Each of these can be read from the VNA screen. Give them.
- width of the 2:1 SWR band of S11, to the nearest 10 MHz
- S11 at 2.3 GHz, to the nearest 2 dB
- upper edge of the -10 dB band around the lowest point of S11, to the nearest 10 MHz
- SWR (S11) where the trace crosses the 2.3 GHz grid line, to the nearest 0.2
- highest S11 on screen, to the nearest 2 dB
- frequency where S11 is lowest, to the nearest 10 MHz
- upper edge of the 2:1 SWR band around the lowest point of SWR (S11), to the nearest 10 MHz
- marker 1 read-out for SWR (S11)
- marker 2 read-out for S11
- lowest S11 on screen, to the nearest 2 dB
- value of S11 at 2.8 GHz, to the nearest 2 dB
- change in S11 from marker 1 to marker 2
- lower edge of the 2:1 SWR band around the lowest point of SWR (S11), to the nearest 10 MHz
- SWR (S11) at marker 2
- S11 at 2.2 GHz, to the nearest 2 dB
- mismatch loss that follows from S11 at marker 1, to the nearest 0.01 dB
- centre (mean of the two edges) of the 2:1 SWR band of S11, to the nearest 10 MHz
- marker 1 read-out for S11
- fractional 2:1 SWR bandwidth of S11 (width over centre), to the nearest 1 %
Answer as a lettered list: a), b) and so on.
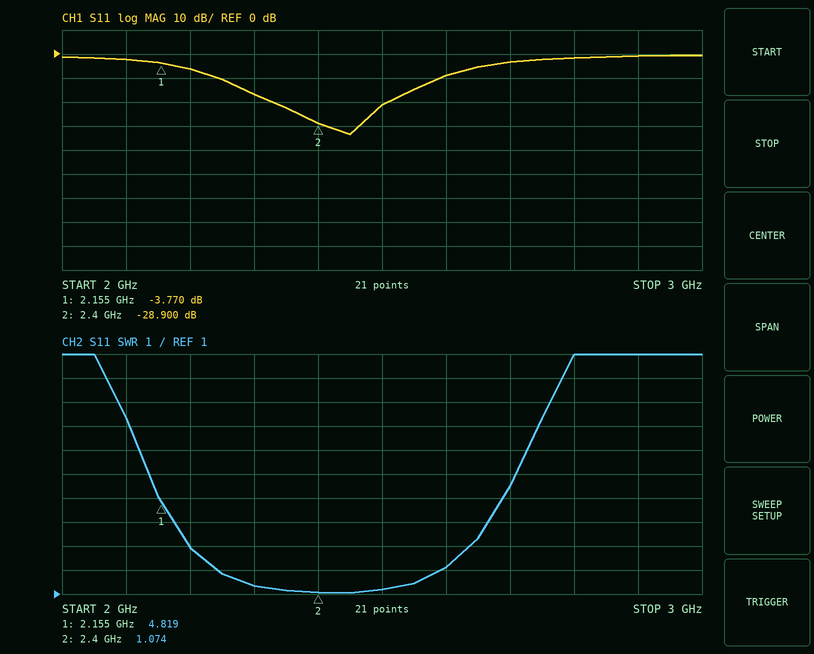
a) 350 MHz
b) -16 dB
c) 2.59 GHz
d) 1.4
e) 0 dB
f) 2.45 GHz
g) 2.59 GHz
h) 4.819
i) -28.900 dB
j) -34 dB
k) -2 dB
l) -25.130 dB
m) 2.24 GHz
n) 1.074
o) -6 dB
p) 2.36 dB
q) 2.42 GHz
r) -3.770 dB
s) 14 %
